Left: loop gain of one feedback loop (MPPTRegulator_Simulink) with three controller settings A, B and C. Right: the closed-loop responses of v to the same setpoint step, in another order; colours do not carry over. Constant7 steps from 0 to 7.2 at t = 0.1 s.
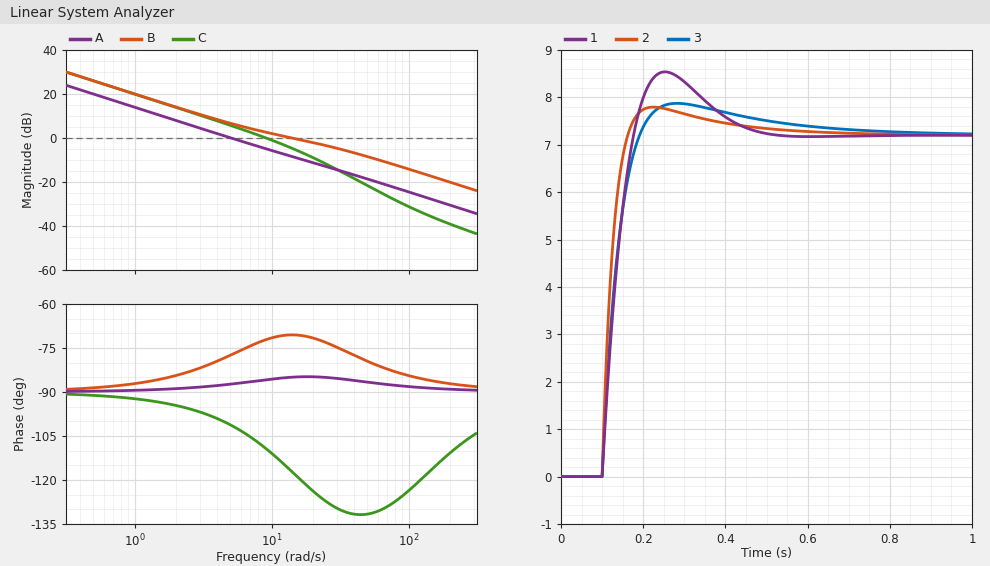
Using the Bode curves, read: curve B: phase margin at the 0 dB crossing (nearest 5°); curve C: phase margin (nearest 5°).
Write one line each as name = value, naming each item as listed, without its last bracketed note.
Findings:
curve B: phase margin at the 0 dB crossing = 110°
curve C: phase margin = 70°
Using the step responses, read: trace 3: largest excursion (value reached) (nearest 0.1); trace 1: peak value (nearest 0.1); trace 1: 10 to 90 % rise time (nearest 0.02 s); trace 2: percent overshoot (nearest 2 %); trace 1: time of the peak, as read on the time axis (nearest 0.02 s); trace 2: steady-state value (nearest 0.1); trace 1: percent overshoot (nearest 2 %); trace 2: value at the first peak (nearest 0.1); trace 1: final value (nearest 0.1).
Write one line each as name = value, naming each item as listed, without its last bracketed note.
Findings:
trace 3: largest excursion (value reached) = 7.9
trace 1: peak value = 8.5
trace 1: 10 to 90 % rise time = 0.06 s
trace 2: percent overshoot = 8 %
trace 1: time of the peak, as read on the time axis = 0.26 s
trace 2: steady-state value = 7.2
trace 1: percent overshoot = 18 %
trace 2: value at the first peak = 7.8
trace 1: final value = 7.2
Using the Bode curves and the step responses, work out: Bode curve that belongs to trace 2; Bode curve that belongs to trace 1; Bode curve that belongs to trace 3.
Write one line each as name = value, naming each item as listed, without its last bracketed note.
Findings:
Bode curve that belongs to trace 2 = B
Bode curve that belongs to trace 1 = C
Bode curve that belongs to trace 3 = A
